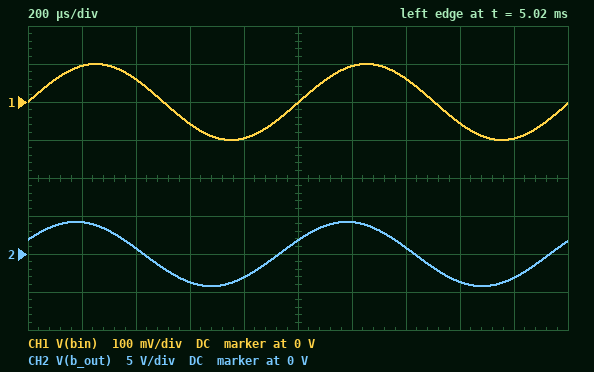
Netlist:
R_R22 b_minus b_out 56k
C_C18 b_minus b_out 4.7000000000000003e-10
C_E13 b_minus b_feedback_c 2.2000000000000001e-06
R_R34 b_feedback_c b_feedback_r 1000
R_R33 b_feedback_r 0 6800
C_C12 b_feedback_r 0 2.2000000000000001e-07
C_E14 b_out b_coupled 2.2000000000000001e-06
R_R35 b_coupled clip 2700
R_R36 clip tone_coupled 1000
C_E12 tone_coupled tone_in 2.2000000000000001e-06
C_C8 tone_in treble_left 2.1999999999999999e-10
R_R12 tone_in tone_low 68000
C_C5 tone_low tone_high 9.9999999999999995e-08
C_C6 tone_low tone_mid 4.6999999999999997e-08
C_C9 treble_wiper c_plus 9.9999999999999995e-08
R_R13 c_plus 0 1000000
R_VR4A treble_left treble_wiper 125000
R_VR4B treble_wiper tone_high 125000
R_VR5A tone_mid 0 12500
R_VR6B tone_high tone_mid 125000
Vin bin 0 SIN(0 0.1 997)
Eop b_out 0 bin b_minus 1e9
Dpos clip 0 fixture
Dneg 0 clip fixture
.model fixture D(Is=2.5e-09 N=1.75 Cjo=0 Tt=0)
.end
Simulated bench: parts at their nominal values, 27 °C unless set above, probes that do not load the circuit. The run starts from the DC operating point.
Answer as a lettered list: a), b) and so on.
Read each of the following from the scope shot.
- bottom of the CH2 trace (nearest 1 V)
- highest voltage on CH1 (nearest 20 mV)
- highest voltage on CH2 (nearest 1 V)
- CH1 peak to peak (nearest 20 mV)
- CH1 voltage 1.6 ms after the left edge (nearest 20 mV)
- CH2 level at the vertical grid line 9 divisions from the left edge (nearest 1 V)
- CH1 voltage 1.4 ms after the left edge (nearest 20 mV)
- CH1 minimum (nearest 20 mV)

a) -4 V
b) 100 mV
c) 4 V
d) 200 mV
e) -60 mV
f) -3 V
g) 60 mV
h) -100 mV
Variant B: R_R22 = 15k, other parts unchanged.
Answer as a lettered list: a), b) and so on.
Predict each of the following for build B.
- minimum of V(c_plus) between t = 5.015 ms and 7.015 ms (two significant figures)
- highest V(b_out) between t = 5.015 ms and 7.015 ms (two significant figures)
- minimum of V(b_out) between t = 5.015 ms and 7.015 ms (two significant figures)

a) -170 mV
b) 1.2 V
c) -1.2 V
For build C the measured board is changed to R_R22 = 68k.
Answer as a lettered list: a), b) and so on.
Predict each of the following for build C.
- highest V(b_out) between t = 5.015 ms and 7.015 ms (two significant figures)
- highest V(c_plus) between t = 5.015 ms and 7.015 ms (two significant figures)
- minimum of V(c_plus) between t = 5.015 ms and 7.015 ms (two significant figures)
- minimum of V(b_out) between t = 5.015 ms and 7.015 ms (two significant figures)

a) 5.1 V
b) 320 mV
c) -320 mV
d) -5.1 V
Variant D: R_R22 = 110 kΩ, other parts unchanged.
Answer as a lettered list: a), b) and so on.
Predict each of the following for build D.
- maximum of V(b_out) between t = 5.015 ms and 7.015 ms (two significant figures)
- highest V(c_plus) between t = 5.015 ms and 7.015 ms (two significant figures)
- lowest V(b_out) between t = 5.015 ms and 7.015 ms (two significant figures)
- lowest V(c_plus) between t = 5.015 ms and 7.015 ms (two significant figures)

a) 7.9 V
b) 360 mV
c) -7.9 V
d) -360 mV
